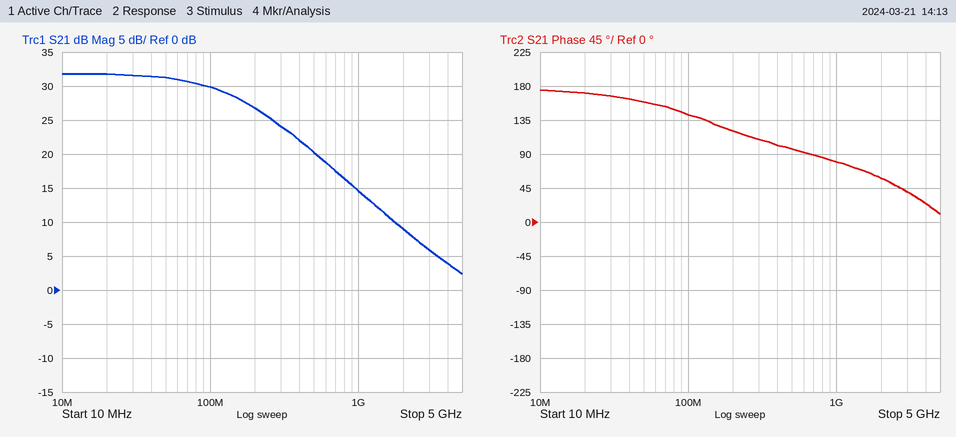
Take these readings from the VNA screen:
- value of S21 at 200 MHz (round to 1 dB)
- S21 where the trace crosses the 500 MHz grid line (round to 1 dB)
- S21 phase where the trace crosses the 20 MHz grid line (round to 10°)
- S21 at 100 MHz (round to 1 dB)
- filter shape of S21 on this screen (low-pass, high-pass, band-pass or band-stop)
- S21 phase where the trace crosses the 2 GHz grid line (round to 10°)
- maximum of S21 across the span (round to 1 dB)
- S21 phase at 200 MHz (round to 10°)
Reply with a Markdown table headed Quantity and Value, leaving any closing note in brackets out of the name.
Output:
| Quantity | Value |
|---|---|
| value of S21 at 200 MHz | 27 dB |
| S21 where the trace crosses the 500 MHz grid line | 20 dB |
| S21 phase where the trace crosses the 20 MHz grid line | 170° |
| S21 at 100 MHz | 30 dB |
| filter shape of S21 on this screen | low-pass |
| S21 phase where the trace crosses the 2 GHz grid line | 60° |
| maximum of S21 across the span | 32 dB |
| S21 phase at 200 MHz | 120° |
